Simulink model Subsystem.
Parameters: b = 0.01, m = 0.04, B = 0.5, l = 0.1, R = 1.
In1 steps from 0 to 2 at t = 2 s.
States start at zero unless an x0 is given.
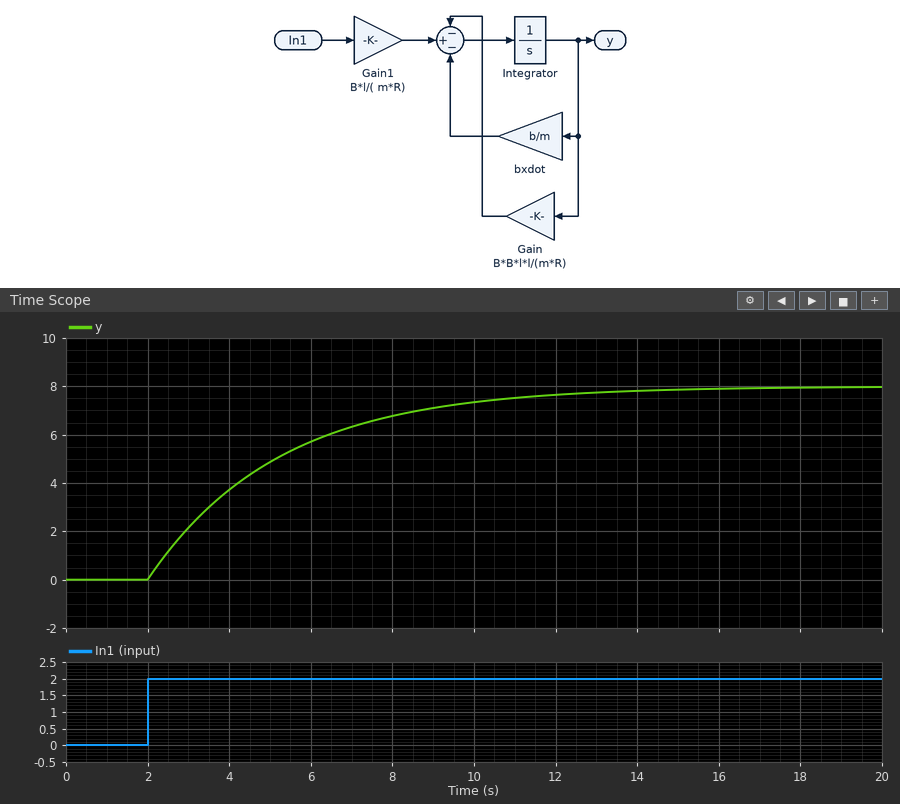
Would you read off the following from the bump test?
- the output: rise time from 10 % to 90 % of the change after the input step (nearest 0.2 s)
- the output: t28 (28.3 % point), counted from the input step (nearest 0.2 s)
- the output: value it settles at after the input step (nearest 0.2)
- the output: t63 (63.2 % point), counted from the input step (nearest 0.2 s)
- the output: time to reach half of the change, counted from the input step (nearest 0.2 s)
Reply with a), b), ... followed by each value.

a) 7.0 s
b) 1.0 s
c) 8.0
d) 3.2 s
e) 2.2 s
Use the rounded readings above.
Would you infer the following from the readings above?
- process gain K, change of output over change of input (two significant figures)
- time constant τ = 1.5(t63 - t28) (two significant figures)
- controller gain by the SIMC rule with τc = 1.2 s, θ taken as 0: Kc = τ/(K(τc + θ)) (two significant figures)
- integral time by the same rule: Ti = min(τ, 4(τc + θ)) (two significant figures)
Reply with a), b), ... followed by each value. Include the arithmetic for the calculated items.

a) (8 - 0) / 2 = 4.0
b) 1.5 × (3.2 - 1) = 3.3 s
c) 3.3 / (4 × (1.2 + 0)) = 0.69
d) min(3.3, 4 × (1.2 + 0)) = 3.3 s
